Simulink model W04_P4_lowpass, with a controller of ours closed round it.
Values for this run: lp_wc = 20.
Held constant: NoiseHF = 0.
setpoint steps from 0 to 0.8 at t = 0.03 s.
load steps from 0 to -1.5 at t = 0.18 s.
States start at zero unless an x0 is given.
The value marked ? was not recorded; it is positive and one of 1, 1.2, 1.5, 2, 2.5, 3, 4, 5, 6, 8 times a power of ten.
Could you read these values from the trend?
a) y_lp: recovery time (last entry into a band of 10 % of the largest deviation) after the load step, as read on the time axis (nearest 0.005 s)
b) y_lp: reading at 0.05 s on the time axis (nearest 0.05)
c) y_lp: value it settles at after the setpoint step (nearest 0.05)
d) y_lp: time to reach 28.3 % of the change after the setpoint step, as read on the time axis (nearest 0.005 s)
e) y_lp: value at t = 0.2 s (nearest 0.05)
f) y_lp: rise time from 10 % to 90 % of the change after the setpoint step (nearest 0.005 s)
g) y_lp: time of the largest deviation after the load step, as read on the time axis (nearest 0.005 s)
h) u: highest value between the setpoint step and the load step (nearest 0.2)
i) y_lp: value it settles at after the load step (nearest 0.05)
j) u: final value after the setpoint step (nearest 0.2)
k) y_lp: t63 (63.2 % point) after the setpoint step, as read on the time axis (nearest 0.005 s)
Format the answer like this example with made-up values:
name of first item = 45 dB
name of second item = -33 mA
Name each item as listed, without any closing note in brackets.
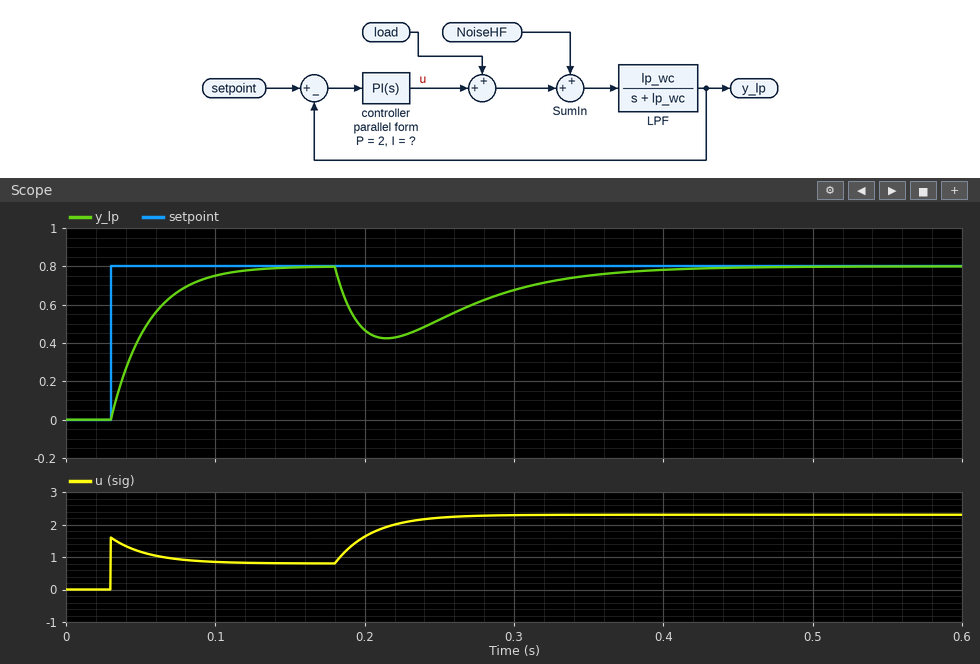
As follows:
y_lp: recovery time (last entry into a band of 10 % of the largest deviation) after the load step, as read on the time axis = 0.365 s
y_lp: reading at 0.05 s on the time axis = 0.45
y_lp: value it settles at after the setpoint step = 0.80
y_lp: time to reach 28.3 % of the change after the setpoint step, as read on the time axis = 0.040 s
y_lp: value at t = 0.2 s = 0.45
y_lp: rise time from 10 % to 90 % of the change after the setpoint step = 0.055 s
y_lp: time of the largest deviation after the load step, as read on the time axis = 0.215 s
u: highest value between the setpoint step and the load step = 1.6
y_lp: value it settles at after the load step = 0.80
u: final value after the setpoint step = 0.8
y_lp: t63 (63.2 % point) after the setpoint step, as read on the time axis = 0.055 s
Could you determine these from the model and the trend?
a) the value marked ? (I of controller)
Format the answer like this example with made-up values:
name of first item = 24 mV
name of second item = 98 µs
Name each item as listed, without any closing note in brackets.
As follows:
the value marked ? = 40
